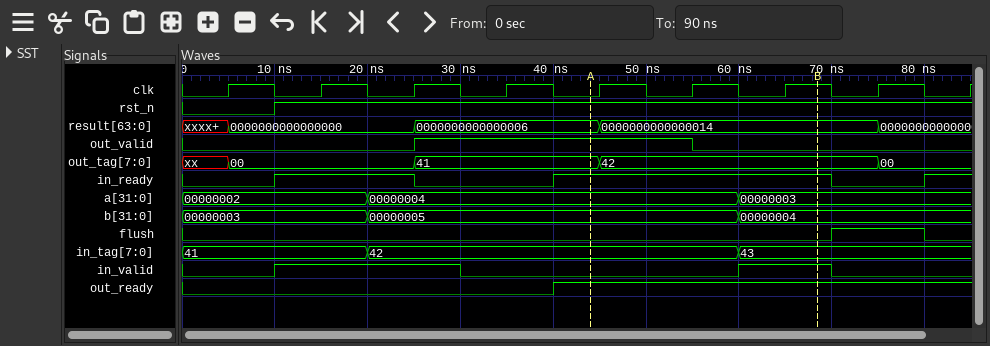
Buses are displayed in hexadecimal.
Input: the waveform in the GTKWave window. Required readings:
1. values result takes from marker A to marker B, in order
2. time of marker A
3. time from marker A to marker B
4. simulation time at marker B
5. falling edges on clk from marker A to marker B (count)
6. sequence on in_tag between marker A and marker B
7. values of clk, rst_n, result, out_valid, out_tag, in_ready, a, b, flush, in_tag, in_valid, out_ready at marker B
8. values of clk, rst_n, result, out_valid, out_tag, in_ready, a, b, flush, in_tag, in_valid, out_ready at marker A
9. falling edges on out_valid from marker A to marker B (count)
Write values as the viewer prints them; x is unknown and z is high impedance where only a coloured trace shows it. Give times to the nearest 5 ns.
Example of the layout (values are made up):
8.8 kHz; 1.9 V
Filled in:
0000000000000006, 0000000000000014; 45 ns; 25 ns; 70 ns; 2; 42, 43; clk=1, rst_n=1, result=0000000000000014, out_valid=0, out_tag=42, in_ready=1, a=00000003, b=00000004, flush=0, in_tag=43, in_valid=1, out_ready=1; clk=0, rst_n=1, result=0000000000000006, out_valid=1, out_tag=41, in_ready=1, a=00000004, b=00000005, flush=0, in_tag=42, in_valid=0, out_ready=1; 1
